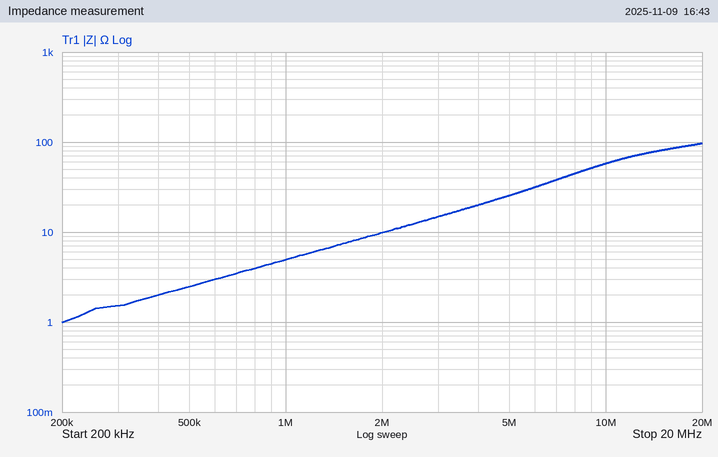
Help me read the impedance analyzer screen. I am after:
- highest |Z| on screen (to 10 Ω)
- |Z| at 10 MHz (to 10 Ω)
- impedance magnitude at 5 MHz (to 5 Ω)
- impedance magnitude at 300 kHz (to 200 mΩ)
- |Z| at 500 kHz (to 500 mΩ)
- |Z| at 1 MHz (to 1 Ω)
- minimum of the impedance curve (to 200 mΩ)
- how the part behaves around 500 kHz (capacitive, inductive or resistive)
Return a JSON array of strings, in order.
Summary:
["100 Ω", "60 Ω", "25 Ω", "1.6 Ω", "2.5 Ω", "5 Ω", "1.0 Ω", "inductive"]
